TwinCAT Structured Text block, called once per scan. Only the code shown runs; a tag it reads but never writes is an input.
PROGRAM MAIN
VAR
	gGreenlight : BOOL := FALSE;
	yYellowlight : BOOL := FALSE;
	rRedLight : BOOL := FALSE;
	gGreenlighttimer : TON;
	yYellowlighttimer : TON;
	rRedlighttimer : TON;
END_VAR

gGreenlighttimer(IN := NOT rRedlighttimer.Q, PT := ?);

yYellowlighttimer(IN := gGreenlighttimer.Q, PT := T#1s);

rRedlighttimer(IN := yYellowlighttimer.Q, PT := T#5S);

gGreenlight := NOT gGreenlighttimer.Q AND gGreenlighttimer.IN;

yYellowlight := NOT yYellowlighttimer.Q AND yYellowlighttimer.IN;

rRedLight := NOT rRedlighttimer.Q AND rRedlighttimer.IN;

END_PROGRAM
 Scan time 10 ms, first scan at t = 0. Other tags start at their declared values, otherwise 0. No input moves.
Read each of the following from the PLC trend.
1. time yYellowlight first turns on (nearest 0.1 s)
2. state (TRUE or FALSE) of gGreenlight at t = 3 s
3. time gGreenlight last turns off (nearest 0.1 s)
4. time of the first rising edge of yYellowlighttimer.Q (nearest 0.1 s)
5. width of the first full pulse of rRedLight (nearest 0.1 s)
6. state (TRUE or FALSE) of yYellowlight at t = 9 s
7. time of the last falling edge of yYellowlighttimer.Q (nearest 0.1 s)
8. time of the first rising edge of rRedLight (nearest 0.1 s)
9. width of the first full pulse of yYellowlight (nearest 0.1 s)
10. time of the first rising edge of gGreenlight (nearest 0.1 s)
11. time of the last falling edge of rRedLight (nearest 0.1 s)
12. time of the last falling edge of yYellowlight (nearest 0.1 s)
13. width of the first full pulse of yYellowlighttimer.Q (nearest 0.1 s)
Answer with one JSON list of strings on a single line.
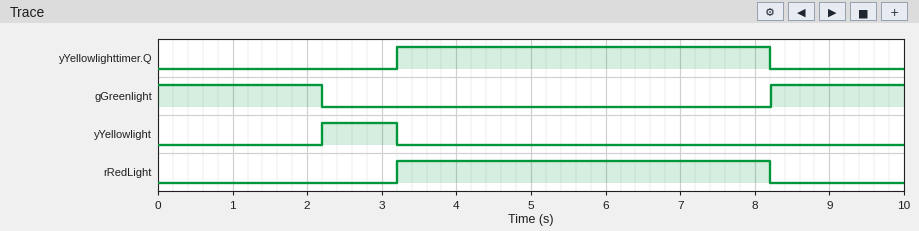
["2.2 s", "FALSE", "2.2 s", "3.2 s", "5.0 s", "FALSE", "8.2 s", "3.2 s", "1.0 s", "8.2 s", "8.2 s", "3.2 s", "5.0 s"]
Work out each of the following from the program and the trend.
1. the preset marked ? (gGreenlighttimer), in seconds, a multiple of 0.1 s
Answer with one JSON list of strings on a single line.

["2.2 s"]
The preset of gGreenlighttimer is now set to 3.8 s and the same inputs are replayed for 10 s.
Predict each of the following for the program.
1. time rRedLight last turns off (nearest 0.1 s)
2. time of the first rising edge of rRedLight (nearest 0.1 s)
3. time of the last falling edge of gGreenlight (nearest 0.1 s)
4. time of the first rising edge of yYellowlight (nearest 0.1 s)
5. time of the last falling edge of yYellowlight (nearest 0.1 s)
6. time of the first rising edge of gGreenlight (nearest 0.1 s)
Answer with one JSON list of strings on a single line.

["9.8 s", "4.8 s", "3.8 s", "3.8 s", "4.8 s", "9.8 s"]
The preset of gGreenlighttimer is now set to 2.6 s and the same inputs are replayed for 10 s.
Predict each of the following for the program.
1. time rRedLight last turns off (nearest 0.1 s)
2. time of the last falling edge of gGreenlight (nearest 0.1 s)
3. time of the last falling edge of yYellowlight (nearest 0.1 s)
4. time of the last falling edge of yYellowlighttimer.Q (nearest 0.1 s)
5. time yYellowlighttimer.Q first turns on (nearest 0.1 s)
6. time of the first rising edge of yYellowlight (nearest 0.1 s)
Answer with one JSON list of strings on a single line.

["8.6 s", "2.6 s", "3.6 s", "8.6 s", "3.6 s", "2.6 s"]
